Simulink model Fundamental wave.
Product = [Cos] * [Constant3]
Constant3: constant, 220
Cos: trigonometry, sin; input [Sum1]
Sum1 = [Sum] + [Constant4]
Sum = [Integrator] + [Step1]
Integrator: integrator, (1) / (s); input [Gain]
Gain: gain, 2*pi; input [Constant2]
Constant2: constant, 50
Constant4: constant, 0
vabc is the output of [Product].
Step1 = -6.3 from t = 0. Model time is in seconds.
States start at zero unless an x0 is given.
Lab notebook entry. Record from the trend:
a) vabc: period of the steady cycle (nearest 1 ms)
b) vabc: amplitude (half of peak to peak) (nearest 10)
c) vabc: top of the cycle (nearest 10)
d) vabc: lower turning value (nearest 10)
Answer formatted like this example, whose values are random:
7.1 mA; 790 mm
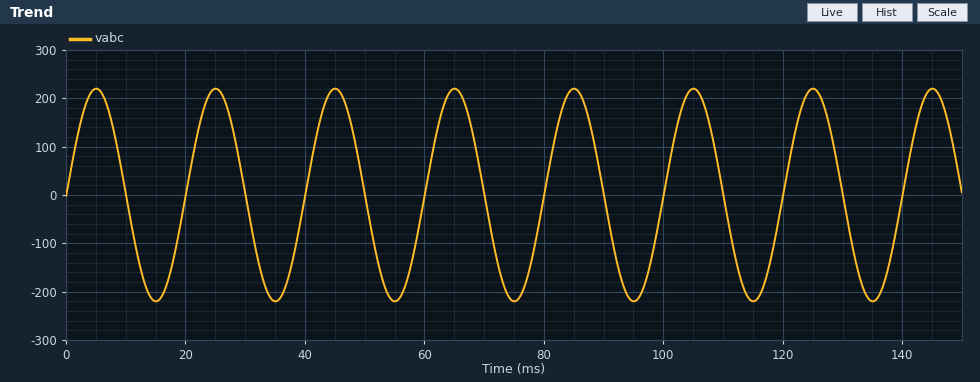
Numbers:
20 ms; 220; 220; -220
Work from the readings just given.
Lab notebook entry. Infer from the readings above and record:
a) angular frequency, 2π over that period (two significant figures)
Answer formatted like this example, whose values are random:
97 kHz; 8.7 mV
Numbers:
0.31 rad/ms
